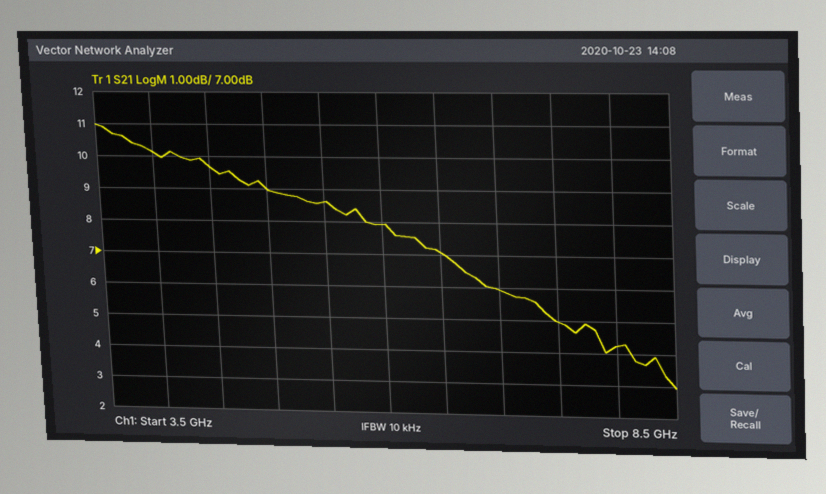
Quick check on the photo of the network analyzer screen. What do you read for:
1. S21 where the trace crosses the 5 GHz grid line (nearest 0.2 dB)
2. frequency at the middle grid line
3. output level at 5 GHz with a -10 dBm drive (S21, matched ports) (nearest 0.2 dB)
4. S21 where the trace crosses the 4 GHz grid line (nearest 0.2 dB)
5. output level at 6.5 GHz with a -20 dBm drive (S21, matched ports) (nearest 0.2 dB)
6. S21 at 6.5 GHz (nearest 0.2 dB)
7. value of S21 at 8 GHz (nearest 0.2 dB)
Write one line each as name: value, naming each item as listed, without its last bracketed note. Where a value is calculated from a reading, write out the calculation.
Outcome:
S21 where the trace crosses the 5 GHz grid line: 9.0 dB
frequency at the middle grid line: 6 GHz
output level at 5 GHz with a -10 dBm drive (S21, matched ports): -10 dBm + (9.0 dB) = -1.0 dBm
S21 where the trace crosses the 4 GHz grid line: 10.2 dB
output level at 6.5 GHz with a -20 dBm drive (S21, matched ports): -20 dBm + (7.0 dB) = -13.0 dBm
S21 at 6.5 GHz: 7.0 dB
value of S21 at 8 GHz: 4.2 dB
